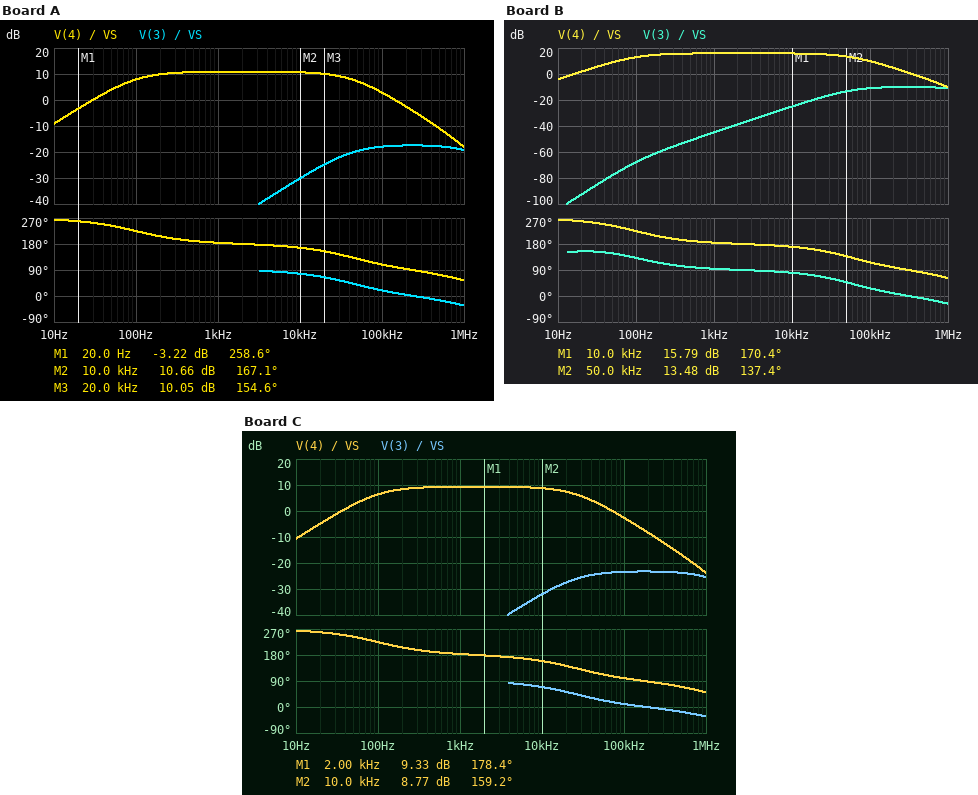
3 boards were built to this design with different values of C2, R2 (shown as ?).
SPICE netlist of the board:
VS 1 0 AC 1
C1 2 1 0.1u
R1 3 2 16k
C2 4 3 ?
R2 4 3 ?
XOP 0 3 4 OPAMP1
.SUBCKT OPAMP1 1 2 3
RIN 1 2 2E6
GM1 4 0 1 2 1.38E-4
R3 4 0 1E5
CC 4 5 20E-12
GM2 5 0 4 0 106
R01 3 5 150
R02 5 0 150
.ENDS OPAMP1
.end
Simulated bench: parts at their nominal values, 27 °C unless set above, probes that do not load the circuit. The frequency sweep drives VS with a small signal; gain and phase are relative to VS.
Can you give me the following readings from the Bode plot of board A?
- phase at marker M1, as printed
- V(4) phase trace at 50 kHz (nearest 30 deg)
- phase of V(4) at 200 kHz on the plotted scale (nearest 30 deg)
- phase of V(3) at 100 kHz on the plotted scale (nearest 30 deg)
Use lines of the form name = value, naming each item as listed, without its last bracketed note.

phase at marker M1, as printed = 258.6 deg
V(4) phase trace at 50 kHz = 120 deg
phase of V(4) at 200 kHz on the plotted scale = 90 deg
phase of V(3) at 100 kHz on the plotted scale = 30 deg
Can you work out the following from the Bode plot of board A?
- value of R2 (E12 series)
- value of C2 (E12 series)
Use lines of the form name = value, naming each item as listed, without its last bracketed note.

value of R2 = 56 kΩ
value of C2 = 56 pF
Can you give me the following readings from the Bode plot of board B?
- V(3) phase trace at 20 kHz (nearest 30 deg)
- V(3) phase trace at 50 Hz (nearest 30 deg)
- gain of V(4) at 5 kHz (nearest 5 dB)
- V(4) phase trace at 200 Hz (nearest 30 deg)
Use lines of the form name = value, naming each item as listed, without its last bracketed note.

V(3) phase trace at 20 kHz = 60 deg
V(3) phase trace at 50 Hz = 150 deg
gain of V(4) at 5 kHz = 15 dB
V(4) phase trace at 200 Hz = 210 deg
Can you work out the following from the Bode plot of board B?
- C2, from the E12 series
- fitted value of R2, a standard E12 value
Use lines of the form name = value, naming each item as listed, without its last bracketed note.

C2, from the E12 series = 18 pF
fitted value of R2, a standard E12 value = 100 kΩ
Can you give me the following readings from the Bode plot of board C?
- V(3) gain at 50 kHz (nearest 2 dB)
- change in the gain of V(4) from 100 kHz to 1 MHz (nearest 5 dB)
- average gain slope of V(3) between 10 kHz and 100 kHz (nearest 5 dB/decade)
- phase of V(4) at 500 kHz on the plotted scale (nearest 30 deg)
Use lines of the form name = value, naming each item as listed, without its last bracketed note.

V(3) gain at 50 kHz = -24 dB
change in the gain of V(4) from 100 kHz to 1 MHz = -20 dB
average gain slope of V(3) between 10 kHz and 100 kHz = 10 dB/decade
phase of V(4) at 500 kHz on the plotted scale = 60 deg
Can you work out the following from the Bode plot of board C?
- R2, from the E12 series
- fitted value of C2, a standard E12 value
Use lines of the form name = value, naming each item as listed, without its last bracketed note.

R2, from the E12 series = 47 kΩ
fitted value of C2, a standard E12 value = 120 pF
